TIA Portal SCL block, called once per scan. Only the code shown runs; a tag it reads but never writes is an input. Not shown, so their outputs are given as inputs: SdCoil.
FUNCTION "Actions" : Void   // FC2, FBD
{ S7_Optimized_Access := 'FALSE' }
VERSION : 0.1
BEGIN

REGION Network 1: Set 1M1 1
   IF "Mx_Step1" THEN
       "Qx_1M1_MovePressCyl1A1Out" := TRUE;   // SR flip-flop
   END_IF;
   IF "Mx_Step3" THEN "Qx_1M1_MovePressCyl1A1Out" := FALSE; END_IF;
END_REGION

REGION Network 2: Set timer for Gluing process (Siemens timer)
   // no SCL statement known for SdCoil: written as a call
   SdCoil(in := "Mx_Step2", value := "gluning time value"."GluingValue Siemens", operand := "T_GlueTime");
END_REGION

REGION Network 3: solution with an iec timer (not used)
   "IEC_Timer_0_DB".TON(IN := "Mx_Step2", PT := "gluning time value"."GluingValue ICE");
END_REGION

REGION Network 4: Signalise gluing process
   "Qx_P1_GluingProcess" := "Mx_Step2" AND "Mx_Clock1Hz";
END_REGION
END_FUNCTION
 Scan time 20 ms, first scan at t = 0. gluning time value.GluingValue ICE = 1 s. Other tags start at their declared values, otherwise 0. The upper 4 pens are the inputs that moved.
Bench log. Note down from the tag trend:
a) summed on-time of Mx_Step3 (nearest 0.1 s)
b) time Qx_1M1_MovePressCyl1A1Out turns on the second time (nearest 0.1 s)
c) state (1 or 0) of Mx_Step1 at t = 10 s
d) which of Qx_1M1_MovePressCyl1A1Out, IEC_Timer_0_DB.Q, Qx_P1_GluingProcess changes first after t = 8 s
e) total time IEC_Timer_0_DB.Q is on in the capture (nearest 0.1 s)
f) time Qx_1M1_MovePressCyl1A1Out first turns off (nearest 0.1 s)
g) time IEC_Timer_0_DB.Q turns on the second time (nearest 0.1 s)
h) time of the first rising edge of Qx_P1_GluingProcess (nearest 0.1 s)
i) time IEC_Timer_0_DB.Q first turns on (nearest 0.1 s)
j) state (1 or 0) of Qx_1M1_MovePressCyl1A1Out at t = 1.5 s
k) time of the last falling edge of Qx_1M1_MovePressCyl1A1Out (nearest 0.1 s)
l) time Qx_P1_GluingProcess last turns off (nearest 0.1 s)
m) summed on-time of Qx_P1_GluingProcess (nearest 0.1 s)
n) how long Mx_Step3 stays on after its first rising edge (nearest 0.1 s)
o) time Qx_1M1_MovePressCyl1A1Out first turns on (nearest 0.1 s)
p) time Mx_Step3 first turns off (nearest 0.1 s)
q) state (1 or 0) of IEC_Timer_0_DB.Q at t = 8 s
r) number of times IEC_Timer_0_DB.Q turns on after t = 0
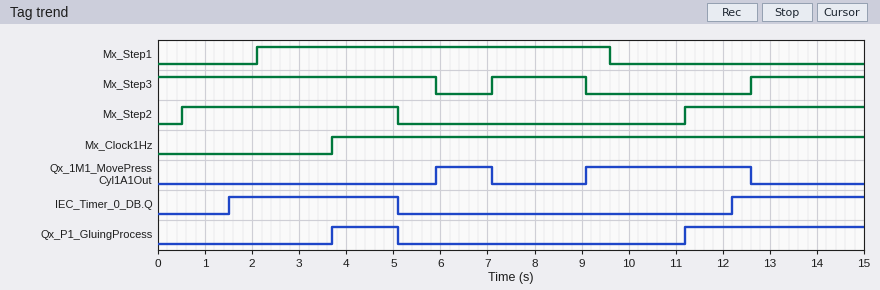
10.3 s
9.1 s
0
Qx_1M1_MovePressCyl1A1Out
6.4 s
7.1 s
12.2 s
3.7 s
1.5 s
0
12.6 s
5.1 s
5.2 s
2.0 s
5.9 s
5.9 s
0
2
